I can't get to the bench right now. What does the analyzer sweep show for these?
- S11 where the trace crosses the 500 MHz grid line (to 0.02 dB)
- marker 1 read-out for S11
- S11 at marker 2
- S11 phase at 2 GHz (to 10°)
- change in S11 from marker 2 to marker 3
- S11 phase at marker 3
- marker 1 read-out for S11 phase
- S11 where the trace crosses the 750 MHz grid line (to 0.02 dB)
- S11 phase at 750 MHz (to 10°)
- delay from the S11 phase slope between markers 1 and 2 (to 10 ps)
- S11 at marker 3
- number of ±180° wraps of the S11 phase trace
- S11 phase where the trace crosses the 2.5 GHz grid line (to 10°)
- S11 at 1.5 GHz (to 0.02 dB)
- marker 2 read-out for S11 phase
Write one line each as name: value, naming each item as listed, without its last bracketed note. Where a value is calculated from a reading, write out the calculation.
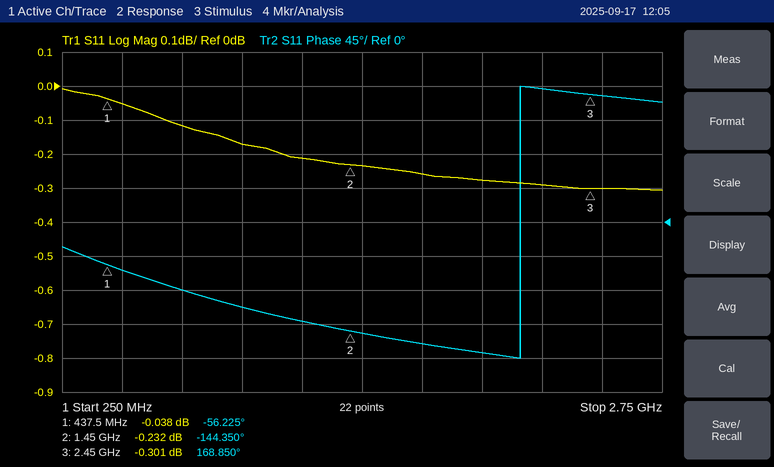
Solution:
S11 where the trace crosses the 500 MHz grid line: -0.06 dB
marker 1 read-out for S11: -0.038 dB
S11 at marker 2: -0.232 dB
S11 phase at 2 GHz: -170°
change in S11 from marker 2 to marker 3: -0.301 − (-0.232) = -0.069 dB
S11 phase at marker 3: 168.850°
marker 1 read-out for S11 phase: -56.225°
S11 where the trace crosses the 750 MHz grid line: -0.12 dB
S11 phase at 750 MHz: -90°
delay from the S11 phase slope between markers 1 and 2: −(-144.35° − (-56.225°))/(360° × 1.0125 GHz) ≈ 242 ps, so 240 ps to the nearest 10 ps
S11 at marker 3: -0.301 dB
number of ±180° wraps of the S11 phase trace: 1
S11 phase where the trace crosses the 2.5 GHz grid line: 170°
S11 at 1.5 GHz: -0.24 dB
marker 2 read-out for S11 phase: -144.350°
